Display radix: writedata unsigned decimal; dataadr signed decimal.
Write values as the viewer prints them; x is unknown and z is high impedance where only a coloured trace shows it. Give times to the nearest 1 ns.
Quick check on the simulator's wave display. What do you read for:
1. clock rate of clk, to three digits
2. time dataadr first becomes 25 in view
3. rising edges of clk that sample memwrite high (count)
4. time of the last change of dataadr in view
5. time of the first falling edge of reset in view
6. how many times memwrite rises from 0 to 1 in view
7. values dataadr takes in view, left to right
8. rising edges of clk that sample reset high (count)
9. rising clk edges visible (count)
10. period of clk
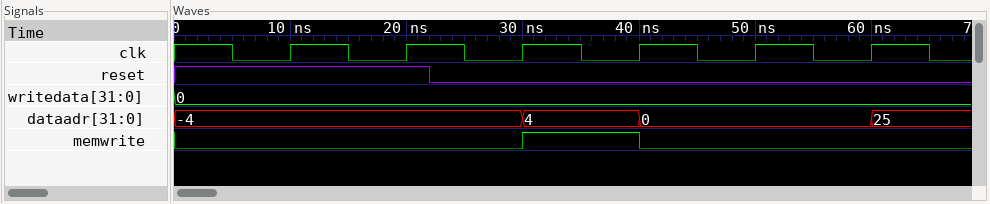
100 MHz
60 ns
1
60 ns
22 ns
1
-4, 4, 0, 25
2
6
10 ns
